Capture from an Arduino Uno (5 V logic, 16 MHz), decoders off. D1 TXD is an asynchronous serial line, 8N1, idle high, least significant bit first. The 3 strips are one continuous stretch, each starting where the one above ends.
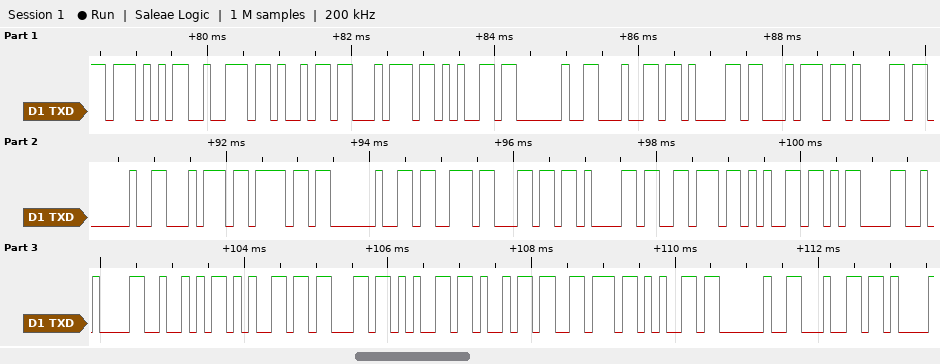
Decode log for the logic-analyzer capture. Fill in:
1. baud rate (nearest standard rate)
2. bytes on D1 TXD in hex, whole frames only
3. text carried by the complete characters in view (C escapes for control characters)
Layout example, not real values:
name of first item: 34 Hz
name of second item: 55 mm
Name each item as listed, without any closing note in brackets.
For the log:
baud rate: 9600 baud
bytes on D1 TXD in hex, whole frames only: 57 72 69 74 65 20 64 61 74 61 20 74 6F 20 73 6C 61 76 65 0D 0A 52 65 63 65 69 76 65 20 64
text carried by the complete characters in view: "Write data to slave\r\nReceive d"
